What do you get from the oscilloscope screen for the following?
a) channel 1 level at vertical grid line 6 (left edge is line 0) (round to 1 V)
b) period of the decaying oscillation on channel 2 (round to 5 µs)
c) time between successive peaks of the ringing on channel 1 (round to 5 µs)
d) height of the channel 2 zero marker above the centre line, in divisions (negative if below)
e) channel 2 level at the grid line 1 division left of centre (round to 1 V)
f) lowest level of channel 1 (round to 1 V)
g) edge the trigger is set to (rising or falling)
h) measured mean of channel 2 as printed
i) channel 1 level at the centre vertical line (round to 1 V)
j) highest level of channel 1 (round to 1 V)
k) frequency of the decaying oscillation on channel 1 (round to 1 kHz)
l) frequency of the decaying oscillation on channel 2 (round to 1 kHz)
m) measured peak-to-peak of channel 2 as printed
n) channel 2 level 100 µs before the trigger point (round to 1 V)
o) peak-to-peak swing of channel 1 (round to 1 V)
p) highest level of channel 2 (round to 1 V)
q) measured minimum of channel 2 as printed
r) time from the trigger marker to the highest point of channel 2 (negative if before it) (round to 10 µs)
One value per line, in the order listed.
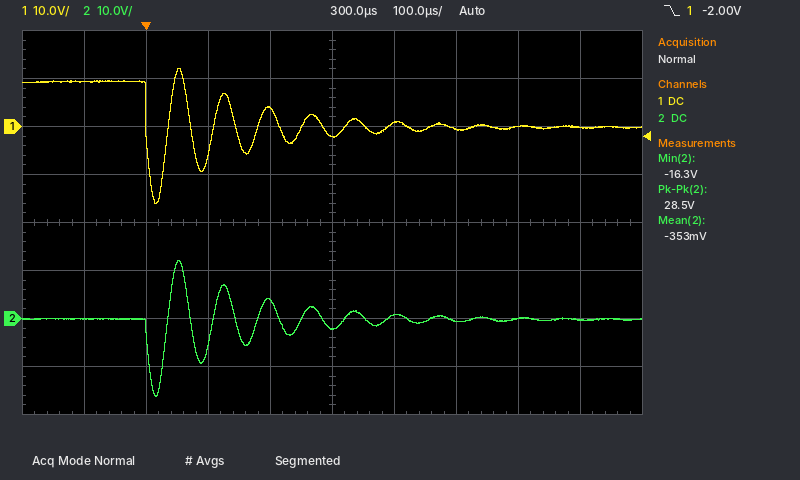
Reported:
1 V
70 µs
70 µs
-2.0 div
4 V
-16 V
falling
-353 mV
-2 V
12 V
14 kHz
14 kHz
28.5 V
0 V
28 V
12 V
-16.3 V
+50 µs
